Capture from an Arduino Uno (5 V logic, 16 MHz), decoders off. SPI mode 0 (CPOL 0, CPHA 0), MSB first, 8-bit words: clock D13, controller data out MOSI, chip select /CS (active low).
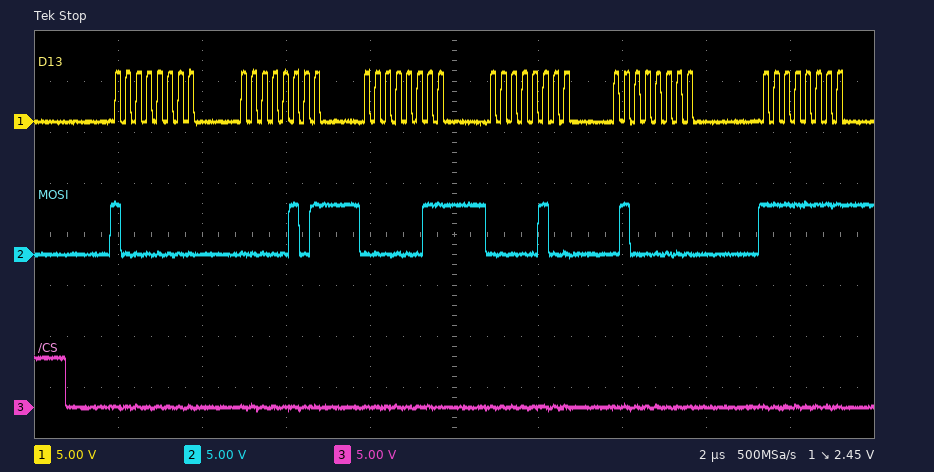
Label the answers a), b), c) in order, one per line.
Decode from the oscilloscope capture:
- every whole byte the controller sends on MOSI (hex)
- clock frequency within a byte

a) 80 05 03 04 40 FF
b) 4 MHz
